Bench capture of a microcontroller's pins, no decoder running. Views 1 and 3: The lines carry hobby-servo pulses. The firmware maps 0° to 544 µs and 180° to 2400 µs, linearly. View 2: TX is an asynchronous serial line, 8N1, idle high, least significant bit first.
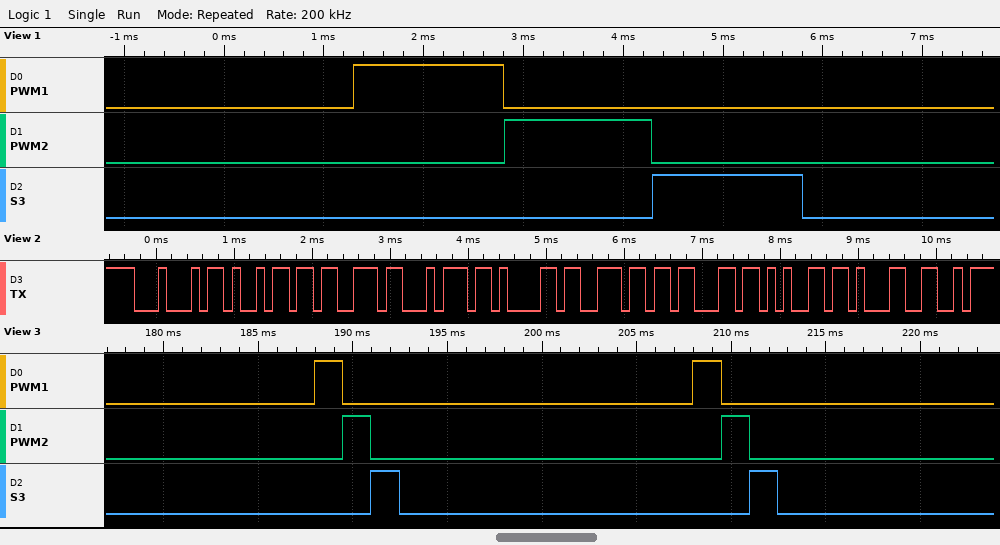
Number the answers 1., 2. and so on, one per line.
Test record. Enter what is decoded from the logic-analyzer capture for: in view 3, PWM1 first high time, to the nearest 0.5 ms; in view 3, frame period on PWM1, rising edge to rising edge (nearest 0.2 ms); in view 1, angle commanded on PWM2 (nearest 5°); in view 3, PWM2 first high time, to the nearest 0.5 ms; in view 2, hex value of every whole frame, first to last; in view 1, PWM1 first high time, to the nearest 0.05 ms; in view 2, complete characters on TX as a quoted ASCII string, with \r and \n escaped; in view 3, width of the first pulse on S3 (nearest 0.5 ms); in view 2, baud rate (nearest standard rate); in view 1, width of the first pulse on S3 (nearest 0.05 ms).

1. 1.5 ms
2. 20.0 ms
3. 90°
4. 1.5 ms
5. 44 69 73 74 61 6E 63 65 31
6. 1.50 ms
7. "Distance1"
8. 1.5 ms
9. 9600 baud
10. 1.50 ms
